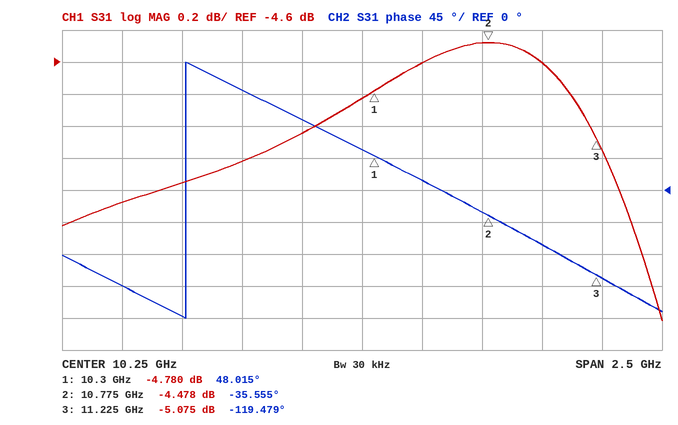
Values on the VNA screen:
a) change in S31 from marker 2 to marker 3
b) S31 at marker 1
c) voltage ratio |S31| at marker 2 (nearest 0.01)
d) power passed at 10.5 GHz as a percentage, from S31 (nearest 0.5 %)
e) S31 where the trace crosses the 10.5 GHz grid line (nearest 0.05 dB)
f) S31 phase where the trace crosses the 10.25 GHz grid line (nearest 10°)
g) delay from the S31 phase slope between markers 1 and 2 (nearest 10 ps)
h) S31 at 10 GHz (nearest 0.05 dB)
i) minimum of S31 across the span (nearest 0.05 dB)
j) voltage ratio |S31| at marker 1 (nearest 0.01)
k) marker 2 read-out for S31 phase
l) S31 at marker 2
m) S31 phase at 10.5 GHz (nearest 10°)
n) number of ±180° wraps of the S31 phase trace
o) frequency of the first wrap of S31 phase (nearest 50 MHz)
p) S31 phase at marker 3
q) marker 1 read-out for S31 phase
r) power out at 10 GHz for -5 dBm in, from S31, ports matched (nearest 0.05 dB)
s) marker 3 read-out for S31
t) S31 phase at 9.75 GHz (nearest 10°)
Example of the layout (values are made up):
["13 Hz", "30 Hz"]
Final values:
["-0.597 dB", "-4.780 dB", "0.60", "34.5 %", "-4.60 dB", "60°", "490 ps", "-5.05 dB", "-6.20 dB", "0.58", "-35.555°", "-4.478 dB", "10°", "1", "9.50 GHz", "-119.479°", "48.015°", "-10.05 dBm", "-5.075 dB", "140°"]
